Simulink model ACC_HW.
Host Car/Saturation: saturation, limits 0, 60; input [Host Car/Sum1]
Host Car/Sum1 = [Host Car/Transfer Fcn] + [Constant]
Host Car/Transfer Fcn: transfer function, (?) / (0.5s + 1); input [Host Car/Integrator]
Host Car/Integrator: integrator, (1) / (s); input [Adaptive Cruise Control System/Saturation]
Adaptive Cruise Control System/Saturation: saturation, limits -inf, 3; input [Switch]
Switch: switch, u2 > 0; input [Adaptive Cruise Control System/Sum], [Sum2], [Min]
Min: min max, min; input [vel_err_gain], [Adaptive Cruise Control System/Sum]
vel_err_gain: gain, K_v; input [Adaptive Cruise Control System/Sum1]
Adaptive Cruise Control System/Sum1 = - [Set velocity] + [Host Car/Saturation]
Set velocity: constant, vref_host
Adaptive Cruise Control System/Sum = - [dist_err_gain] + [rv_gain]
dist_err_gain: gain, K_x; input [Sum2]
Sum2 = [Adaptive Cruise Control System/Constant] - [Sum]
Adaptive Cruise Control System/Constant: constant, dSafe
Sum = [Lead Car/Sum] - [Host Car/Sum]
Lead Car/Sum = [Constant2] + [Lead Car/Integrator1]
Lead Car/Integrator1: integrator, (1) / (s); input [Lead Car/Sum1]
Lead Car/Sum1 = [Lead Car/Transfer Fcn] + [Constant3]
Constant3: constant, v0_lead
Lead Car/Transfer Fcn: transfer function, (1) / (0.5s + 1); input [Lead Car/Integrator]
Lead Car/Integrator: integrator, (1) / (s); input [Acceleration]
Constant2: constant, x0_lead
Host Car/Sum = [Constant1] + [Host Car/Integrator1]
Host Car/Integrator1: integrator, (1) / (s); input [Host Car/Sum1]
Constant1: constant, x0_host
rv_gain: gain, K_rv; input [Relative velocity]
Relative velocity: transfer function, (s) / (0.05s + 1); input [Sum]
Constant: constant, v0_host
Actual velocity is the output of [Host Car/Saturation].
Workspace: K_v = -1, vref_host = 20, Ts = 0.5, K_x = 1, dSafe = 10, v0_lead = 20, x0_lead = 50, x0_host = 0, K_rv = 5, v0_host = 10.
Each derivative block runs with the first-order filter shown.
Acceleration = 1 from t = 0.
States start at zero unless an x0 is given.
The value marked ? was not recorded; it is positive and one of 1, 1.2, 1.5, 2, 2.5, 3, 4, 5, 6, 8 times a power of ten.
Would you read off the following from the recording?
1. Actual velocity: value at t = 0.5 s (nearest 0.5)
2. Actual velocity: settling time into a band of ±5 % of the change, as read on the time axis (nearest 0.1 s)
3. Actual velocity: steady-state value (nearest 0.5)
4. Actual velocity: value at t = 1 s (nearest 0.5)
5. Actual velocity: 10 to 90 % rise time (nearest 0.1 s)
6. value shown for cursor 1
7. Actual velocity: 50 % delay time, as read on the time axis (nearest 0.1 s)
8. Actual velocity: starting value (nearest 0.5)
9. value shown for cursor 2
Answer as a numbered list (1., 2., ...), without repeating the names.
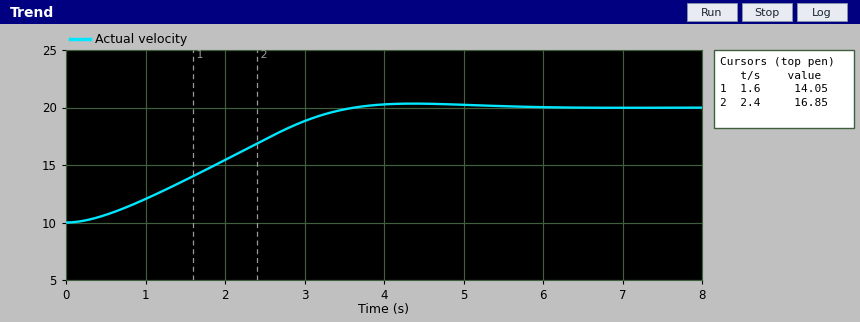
1. 10.5
2. 3.3 s
3. 20.0
4. 12.0
5. 2.4 s
6. 14.05
7. 1.9 s
8. 10.0
9. 16.85
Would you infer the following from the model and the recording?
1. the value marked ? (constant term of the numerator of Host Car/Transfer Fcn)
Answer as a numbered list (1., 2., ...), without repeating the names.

1. 1.2
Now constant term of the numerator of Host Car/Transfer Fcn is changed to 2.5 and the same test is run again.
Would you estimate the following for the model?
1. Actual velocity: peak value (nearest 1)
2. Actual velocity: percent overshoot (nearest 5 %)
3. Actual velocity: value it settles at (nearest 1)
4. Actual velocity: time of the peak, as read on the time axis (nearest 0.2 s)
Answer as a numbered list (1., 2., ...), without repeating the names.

1. 21
2. 10 %
3. 20
4. 2.4 s
